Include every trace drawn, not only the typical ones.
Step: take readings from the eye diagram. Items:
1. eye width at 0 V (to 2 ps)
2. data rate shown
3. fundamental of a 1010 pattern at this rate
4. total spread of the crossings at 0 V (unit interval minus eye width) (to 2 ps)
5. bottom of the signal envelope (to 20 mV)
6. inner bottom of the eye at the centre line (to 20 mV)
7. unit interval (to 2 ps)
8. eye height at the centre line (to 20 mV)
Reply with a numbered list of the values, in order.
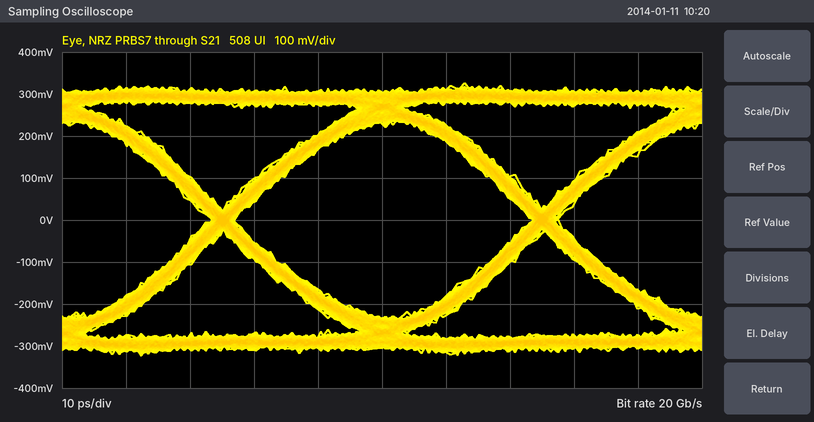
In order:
1. 46 ps
2. 20 Gb/s
3. 10 GHz
4. 4 ps
5. -320 mV
6. -240 mV
7. 50 ps
8. 460 mV
